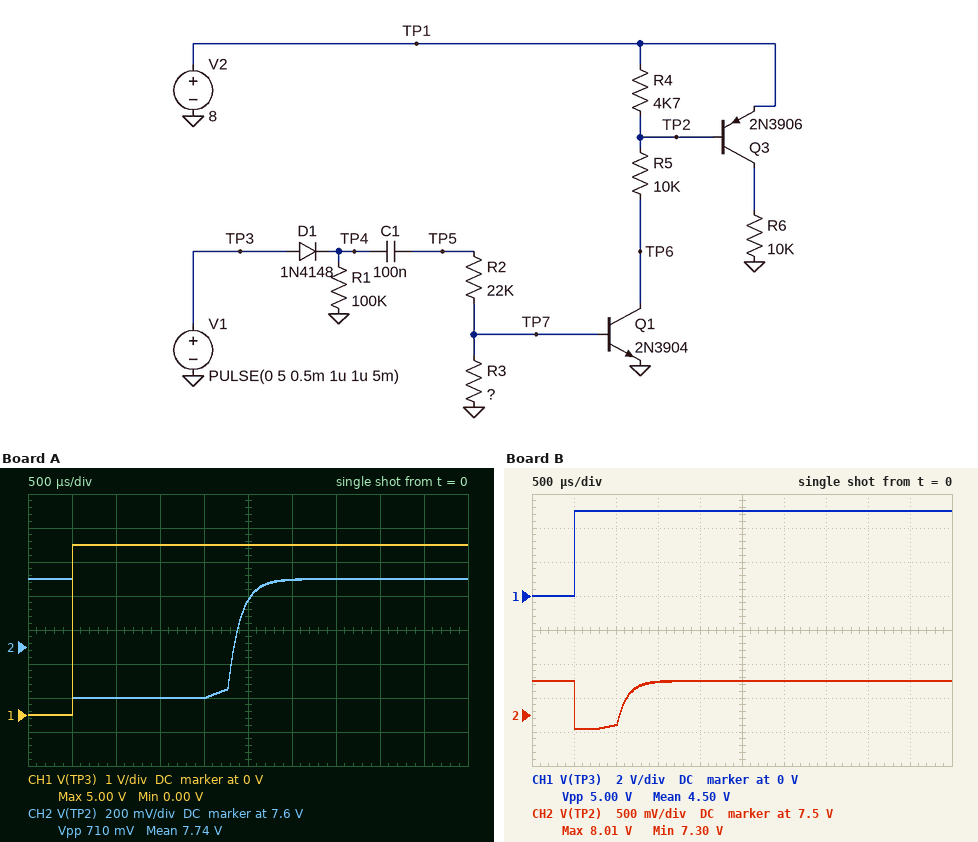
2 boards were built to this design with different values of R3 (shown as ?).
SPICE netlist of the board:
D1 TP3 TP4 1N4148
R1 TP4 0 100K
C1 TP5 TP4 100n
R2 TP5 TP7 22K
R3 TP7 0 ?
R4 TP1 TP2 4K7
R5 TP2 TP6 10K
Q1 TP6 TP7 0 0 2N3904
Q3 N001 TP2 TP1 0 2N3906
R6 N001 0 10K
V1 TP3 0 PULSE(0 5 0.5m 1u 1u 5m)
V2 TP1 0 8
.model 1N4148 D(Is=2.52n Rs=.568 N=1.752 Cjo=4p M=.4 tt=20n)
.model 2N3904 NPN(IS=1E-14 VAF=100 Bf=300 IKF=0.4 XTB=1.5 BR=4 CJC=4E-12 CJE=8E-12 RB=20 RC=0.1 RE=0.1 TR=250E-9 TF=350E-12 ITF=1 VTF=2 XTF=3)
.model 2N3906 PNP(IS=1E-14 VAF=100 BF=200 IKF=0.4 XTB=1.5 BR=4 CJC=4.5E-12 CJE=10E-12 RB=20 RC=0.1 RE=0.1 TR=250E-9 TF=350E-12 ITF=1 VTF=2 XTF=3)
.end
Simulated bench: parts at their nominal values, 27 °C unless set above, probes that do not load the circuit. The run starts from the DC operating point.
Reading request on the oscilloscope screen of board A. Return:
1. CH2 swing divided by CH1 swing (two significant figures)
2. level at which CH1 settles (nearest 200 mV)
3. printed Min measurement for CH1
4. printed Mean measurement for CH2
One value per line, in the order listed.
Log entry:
0.14
5.0 V
0.00 V
7.74 V
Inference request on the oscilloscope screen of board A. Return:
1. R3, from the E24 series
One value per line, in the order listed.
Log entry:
7.5 kΩ
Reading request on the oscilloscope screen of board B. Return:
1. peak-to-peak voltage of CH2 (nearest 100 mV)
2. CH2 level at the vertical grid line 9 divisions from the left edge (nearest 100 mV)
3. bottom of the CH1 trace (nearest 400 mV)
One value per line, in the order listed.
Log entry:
700 mV
8.0 V
0 V
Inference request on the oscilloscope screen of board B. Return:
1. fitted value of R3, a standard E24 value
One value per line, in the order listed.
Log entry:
4.3 kΩ
